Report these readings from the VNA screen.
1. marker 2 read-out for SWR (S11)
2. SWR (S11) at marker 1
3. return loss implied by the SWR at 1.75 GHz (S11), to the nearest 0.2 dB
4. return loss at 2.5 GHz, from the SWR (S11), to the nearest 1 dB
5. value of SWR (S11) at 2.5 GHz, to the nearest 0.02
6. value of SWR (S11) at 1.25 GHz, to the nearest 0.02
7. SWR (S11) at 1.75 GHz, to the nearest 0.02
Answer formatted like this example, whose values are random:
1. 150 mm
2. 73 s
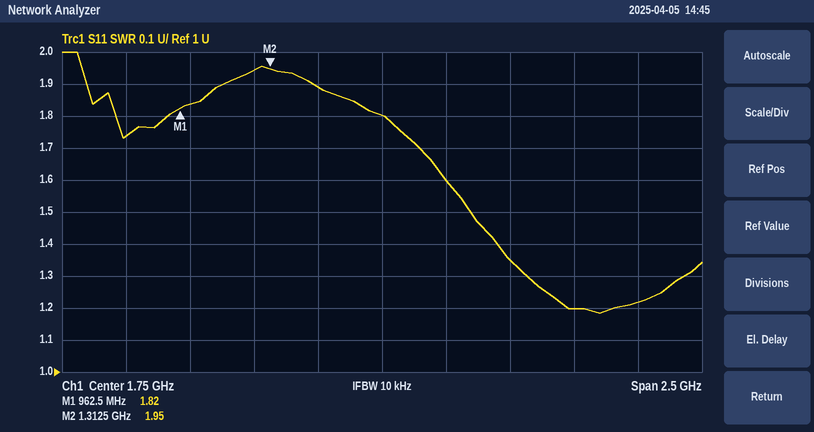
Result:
1. 1.95
2. 1.82
3. 10.8 dB
4. 21 dB
5. 1.20
6. 1.94
7. 1.80
